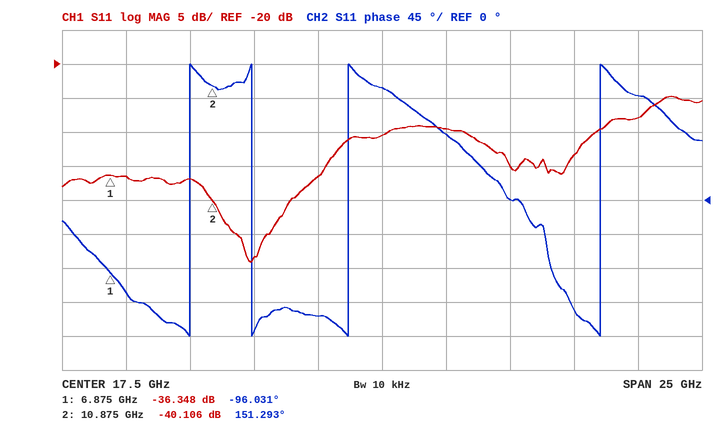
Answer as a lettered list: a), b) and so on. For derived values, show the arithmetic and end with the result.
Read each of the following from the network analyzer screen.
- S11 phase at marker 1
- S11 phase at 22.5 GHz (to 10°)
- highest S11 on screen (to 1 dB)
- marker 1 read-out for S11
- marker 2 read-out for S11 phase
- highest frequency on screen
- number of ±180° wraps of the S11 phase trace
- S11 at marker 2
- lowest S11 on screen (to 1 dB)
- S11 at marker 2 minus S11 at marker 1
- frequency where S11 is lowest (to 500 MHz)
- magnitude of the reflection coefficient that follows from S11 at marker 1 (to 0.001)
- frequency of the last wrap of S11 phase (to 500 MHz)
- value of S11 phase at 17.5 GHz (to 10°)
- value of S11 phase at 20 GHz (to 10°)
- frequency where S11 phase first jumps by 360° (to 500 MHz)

a) -96.031°
b) 0°
c) -25 dB
d) -36.348 dB
e) 151.293°
f) 30 GHz
g) 4
h) -40.106 dB
i) -49 dB
j) -40.106 − (-36.348) = -3.758 dB
k) 12.5 GHz
l) 10^(-36.348/20) ≈ 0.015
m) 26.0 GHz
n) 150°
o) 90°
p) 10.0 GHz
